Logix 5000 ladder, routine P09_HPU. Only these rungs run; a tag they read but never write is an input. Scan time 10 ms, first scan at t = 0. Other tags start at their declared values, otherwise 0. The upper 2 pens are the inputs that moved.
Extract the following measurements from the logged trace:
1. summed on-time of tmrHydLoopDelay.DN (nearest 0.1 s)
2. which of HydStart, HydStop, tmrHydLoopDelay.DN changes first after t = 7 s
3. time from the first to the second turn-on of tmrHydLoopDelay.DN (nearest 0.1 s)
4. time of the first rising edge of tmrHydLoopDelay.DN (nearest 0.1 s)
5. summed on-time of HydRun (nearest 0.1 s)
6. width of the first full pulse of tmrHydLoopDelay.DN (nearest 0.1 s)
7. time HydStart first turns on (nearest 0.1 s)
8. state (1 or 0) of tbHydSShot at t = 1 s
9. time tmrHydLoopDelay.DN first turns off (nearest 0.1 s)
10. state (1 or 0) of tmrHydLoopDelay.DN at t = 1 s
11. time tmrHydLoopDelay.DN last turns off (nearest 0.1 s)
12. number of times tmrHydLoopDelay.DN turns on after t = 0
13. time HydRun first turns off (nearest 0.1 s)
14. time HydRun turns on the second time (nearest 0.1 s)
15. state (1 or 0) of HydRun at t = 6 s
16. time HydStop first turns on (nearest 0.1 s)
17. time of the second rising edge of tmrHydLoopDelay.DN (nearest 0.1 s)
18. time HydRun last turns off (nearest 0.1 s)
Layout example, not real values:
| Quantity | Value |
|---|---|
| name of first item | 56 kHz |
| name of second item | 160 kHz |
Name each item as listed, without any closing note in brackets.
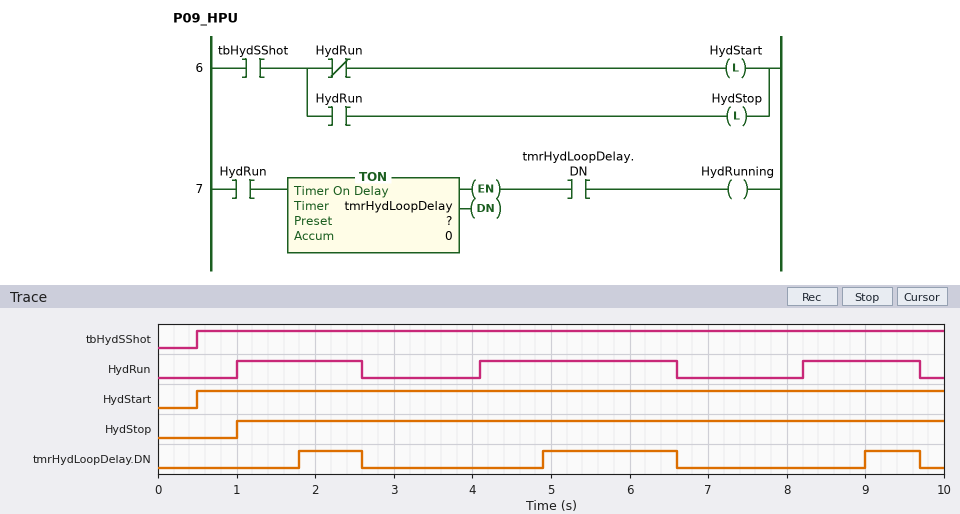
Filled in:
| Quantity | Value |
|---|---|
| summed on-time of tmrHydLoopDelay.DN | 3.2 s |
| which of HydStart, HydStop, tmrHydLoopDelay.DN changes first after t = 7 s | tmrHydLoopDelay.DN |
| time from the first to the second turn-on of tmrHydLoopDelay.DN | 3.1 s |
| time of the first rising edge of tmrHydLoopDelay.DN | 1.8 s |
| summed on-time of HydRun | 5.6 s |
| width of the first full pulse of tmrHydLoopDelay.DN | 0.8 s |
| time HydStart first turns on | 0.5 s |
| state (1 or 0) of tbHydSShot at t = 1 s | 1 |
| time tmrHydLoopDelay.DN first turns off | 2.6 s |
| state (1 or 0) of tmrHydLoopDelay.DN at t = 1 s | 0 |
| time tmrHydLoopDelay.DN last turns off | 9.7 s |
| number of times tmrHydLoopDelay.DN turns on after t = 0 | 3 |
| time HydRun first turns off | 2.6 s |
| time HydRun turns on the second time | 4.1 s |
| state (1 or 0) of HydRun at t = 6 s | 1 |
| time HydStop first turns on | 1.0 s |
| time of the second rising edge of tmrHydLoopDelay.DN | 4.9 s |
| time HydRun last turns off | 9.7 s |
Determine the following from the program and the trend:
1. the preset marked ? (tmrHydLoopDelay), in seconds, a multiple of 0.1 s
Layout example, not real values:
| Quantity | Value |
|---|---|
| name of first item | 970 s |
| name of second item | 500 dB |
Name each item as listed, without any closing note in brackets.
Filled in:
| Quantity | Value |
|---|---|
| the preset marked ? (tmrHydLoopDelay), in seconds, a multiple of 0.1 s | 0.8 s |
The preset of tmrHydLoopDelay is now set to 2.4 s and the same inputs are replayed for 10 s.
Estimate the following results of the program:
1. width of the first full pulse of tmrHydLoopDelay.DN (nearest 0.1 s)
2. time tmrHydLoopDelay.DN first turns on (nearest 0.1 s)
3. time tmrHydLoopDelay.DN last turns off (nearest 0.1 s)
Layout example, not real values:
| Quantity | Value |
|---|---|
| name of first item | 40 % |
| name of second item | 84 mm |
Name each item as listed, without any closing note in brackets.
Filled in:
| Quantity | Value |
|---|---|
| width of the first full pulse of tmrHydLoopDelay.DN | 0.1 s |
| time tmrHydLoopDelay.DN first turns on | 6.5 s |
| time tmrHydLoopDelay.DN last turns off | 6.6 s |
